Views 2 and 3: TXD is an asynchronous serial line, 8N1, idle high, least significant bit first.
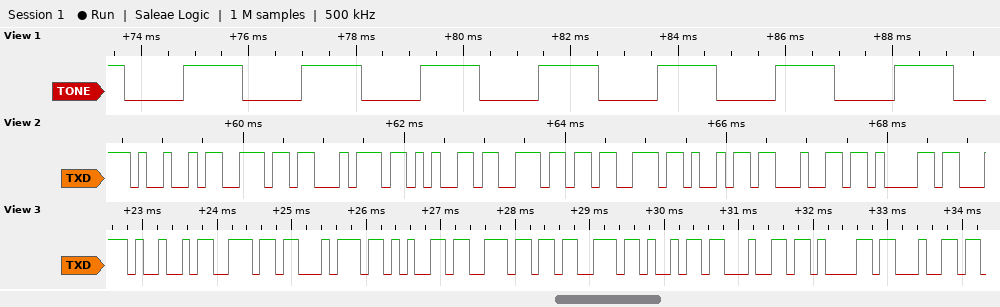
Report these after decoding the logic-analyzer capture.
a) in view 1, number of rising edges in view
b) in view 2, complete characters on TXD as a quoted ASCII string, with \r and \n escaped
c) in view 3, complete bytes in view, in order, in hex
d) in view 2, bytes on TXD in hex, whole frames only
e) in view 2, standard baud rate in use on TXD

7
"Intensida"
49 6E 74 65 6E 73 69 64 61 64
49 6E 74 65 6E 73 69 64 61
9600 baud
